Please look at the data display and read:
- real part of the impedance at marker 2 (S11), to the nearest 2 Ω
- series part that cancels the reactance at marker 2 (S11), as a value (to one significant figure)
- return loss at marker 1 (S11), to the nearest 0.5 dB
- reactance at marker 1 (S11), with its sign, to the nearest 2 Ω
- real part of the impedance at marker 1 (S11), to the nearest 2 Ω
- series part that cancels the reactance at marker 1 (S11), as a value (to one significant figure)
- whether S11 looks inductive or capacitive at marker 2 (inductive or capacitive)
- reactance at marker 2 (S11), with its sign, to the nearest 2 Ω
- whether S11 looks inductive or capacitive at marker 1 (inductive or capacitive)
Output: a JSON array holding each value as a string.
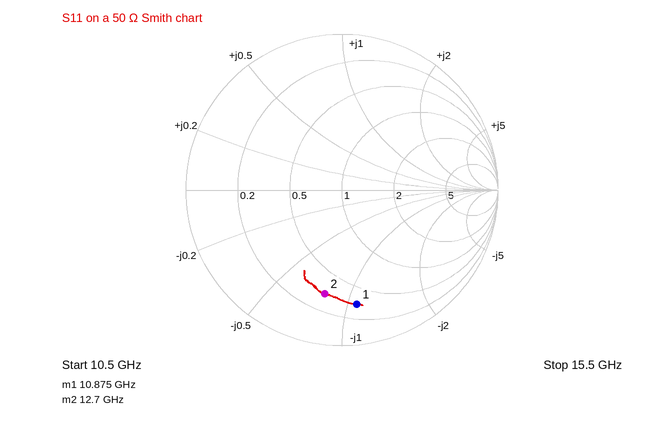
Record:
["16 Ω", "500 pH", "2.5 dB", "-54 Ω", "16 Ω", "800 pH", "capacitive", "-40 Ω", "capacitive"]
